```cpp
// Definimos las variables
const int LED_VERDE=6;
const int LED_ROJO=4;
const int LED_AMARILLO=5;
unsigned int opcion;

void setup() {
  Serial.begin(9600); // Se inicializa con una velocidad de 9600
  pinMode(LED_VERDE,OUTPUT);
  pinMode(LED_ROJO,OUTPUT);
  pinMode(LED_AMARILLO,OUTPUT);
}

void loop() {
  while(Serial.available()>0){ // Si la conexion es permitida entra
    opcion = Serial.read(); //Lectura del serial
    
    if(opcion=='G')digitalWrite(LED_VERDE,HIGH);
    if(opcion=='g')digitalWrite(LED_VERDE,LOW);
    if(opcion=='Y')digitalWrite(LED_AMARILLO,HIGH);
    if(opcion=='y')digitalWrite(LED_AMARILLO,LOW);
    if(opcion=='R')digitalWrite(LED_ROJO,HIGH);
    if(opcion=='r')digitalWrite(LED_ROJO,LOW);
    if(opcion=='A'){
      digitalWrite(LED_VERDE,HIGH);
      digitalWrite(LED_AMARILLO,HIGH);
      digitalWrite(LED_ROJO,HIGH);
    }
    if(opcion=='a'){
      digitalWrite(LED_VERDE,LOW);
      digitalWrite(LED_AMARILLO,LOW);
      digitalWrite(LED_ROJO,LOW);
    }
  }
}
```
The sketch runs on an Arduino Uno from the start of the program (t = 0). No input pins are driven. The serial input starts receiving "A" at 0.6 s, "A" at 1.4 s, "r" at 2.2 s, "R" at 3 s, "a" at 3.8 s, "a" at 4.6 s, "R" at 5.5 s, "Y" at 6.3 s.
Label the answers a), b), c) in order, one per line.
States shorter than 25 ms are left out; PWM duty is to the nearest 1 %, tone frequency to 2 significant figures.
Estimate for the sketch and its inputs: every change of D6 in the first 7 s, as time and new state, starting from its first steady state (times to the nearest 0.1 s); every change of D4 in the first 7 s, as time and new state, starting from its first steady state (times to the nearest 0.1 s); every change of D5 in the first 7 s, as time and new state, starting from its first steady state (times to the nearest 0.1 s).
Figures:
a) 0 s low; 0.6 s high; 3.8 s low
b) 0 s low; 0.6 s high; 2.2 s low; 3 s high; 3.8 s low; 5.5 s high
c) 0 s low; 0.6 s high; 3.8 s low; 6.3 s high
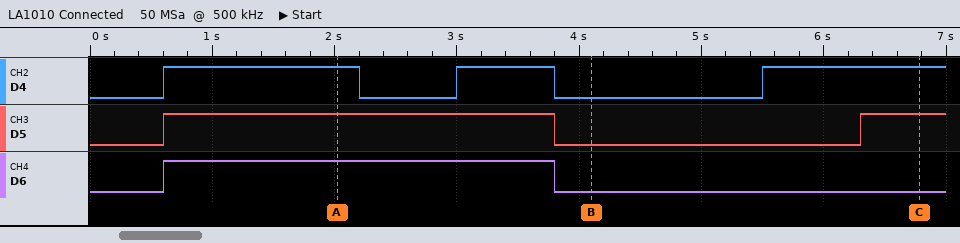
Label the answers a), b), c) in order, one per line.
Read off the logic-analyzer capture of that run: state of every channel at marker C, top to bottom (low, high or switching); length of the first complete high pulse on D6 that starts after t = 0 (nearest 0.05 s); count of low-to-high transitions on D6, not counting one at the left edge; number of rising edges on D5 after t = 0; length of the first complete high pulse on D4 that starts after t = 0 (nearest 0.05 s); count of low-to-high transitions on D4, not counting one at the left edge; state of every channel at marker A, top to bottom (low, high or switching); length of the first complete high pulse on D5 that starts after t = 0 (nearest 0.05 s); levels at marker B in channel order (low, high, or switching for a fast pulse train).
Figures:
a) D4 high, D5 high, D6 low
b) 3.20 s
c) 1
d) 2
e) 1.60 s
f) 3
g) D4 high, D5 high, D6 high
h) 3.20 s
i) D4 low, D5 low, D6 low
